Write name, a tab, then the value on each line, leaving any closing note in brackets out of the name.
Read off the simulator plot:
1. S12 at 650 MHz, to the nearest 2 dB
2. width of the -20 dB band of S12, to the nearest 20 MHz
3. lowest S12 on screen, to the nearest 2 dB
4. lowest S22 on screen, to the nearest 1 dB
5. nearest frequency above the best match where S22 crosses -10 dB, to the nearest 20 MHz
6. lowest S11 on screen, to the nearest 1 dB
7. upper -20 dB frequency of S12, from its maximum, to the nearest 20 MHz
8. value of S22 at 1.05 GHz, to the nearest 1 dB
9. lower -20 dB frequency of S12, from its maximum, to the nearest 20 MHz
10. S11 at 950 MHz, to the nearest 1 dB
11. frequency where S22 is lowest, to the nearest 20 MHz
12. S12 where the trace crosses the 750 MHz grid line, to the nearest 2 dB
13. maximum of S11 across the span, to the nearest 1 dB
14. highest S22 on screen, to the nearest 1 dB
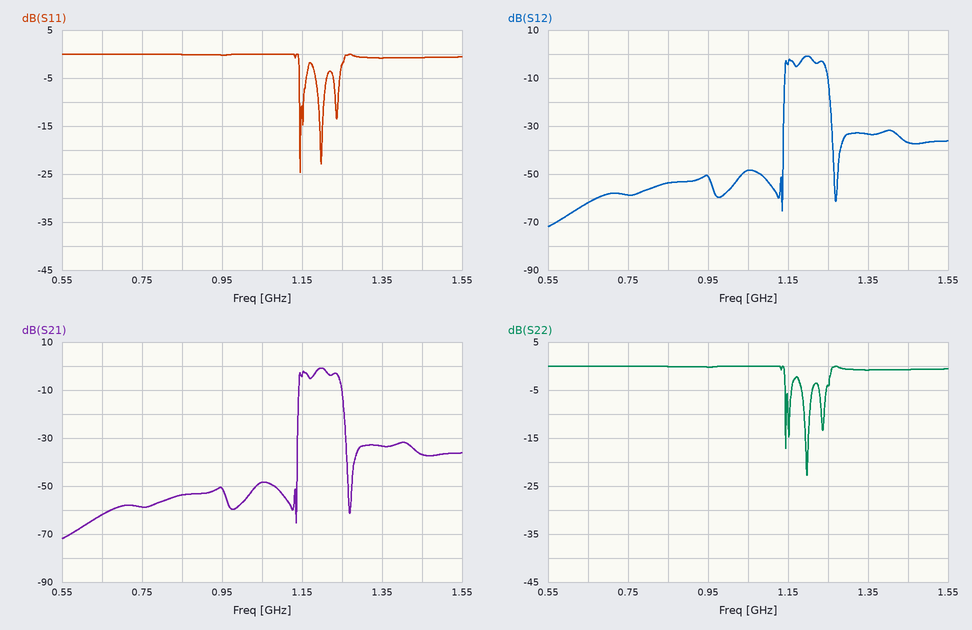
S12 at 650 MHz, to the nearest 2 dB	-62 dB
width of the -20 dB band of S12, to the nearest 20 MHz	120 MHz
lowest S12 on screen, to the nearest 2 dB	-72 dB
lowest S22 on screen, to the nearest 1 dB	-23 dB
nearest frequency above the best match where S22 crosses -10 dB, to the nearest 20 MHz	1.20 GHz
lowest S11 on screen, to the nearest 1 dB	-25 dB
upper -20 dB frequency of S12, from its maximum, to the nearest 20 MHz	1.26 GHz
value of S22 at 1.05 GHz, to the nearest 1 dB	0 dB
lower -20 dB frequency of S12, from its maximum, to the nearest 20 MHz	1.14 GHz
S11 at 950 MHz, to the nearest 1 dB	0 dB
frequency where S22 is lowest, to the nearest 20 MHz	1.20 GHz
S12 where the trace crosses the 750 MHz grid line, to the nearest 2 dB	-58 dB
maximum of S11 across the span, to the nearest 1 dB	0 dB
highest S22 on screen, to the nearest 1 dB	0 dB
